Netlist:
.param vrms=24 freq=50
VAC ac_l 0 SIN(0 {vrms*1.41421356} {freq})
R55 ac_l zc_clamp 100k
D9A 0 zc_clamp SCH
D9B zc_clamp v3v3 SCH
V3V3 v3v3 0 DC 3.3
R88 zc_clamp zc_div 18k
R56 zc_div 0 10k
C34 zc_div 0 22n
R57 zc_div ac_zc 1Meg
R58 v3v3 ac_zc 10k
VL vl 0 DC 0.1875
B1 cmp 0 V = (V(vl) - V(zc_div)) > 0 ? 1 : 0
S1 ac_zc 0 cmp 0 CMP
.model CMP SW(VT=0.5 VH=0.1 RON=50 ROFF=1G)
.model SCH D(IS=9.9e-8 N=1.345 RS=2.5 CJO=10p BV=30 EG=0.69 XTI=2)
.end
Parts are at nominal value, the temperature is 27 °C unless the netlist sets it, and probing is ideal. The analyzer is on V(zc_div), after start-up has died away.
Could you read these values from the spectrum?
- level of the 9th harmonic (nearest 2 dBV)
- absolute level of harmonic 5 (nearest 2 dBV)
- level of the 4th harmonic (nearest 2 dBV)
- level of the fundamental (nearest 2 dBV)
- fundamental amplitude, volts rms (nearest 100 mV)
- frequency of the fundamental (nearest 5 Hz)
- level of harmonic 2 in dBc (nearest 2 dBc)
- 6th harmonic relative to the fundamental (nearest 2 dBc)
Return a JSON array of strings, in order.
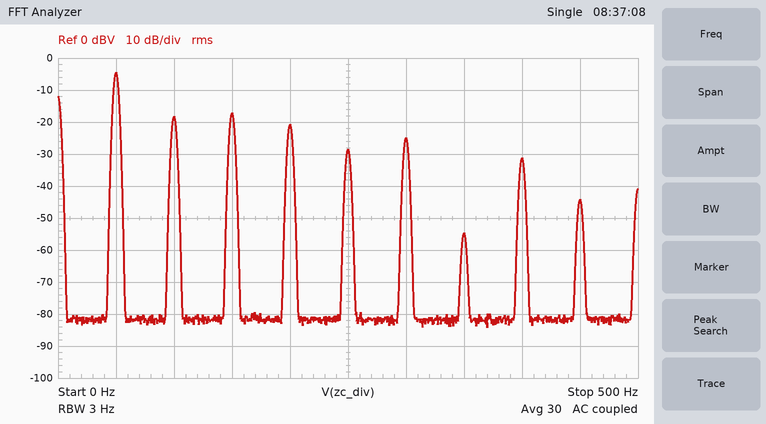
["-44 dBV", "-28 dBV", "-20 dBV", "-4 dBV", "600 mV", "50 Hz", "-14 dBc", "-20 dBc"]
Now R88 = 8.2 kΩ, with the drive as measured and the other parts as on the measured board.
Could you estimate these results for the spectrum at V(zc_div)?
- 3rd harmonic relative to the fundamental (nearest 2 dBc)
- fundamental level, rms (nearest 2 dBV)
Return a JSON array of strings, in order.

["-16 dBc", "-2 dBV"]
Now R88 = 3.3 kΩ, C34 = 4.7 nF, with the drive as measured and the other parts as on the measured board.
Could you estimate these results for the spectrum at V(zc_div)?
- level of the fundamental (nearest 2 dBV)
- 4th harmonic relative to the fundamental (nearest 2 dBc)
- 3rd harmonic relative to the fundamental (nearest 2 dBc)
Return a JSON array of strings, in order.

["0 dBV", "-20 dBc", "-24 dBc"]
